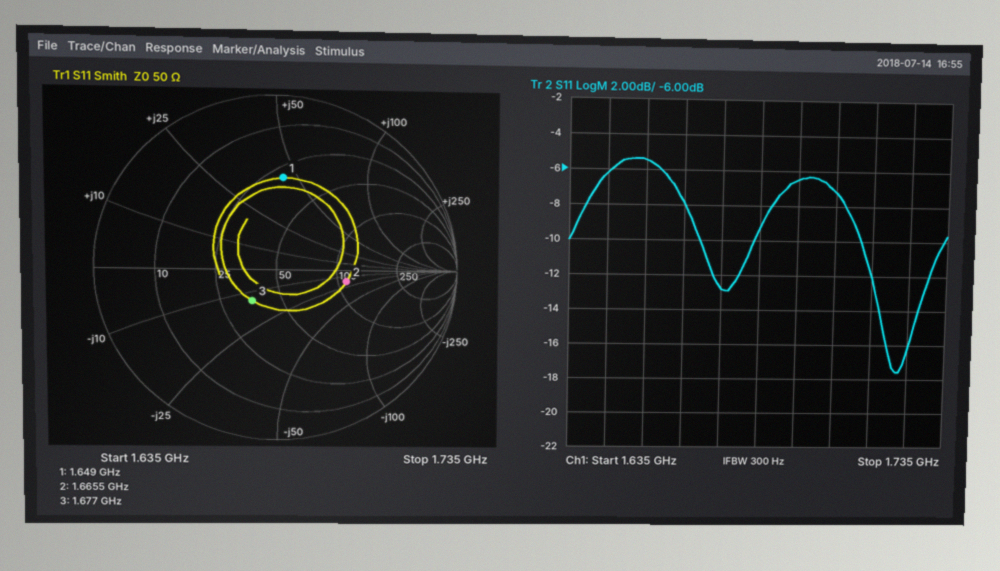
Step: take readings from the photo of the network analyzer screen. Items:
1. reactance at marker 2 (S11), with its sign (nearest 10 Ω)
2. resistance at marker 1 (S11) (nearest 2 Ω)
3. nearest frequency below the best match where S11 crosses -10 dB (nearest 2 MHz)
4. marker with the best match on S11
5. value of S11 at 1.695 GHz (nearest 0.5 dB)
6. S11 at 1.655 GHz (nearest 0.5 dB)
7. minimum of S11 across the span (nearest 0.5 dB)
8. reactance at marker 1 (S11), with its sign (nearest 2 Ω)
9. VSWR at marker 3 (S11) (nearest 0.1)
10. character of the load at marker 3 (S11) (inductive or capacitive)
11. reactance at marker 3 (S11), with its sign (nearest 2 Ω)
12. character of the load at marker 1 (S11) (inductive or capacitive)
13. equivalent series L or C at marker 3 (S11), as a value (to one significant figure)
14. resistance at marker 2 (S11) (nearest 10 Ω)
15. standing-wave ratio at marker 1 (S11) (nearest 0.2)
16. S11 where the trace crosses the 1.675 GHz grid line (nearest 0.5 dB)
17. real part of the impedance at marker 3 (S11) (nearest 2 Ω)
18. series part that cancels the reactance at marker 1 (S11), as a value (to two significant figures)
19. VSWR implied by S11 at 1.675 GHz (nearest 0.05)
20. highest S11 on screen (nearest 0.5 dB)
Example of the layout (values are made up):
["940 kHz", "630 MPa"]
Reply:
["-20 Ω", "30 Ω", "1.712 GHz", "marker 3", "-6.5 dB", "-5.5 dB", "-17.5 dB", "+44 Ω", "1.6", "capacitive", "-14 Ω", "inductive", "7 pF", "110 Ω", "3.2", "-13.0 dB", "36 Ω", "2.2 pF", "1.60", "-5.5 dB"]
